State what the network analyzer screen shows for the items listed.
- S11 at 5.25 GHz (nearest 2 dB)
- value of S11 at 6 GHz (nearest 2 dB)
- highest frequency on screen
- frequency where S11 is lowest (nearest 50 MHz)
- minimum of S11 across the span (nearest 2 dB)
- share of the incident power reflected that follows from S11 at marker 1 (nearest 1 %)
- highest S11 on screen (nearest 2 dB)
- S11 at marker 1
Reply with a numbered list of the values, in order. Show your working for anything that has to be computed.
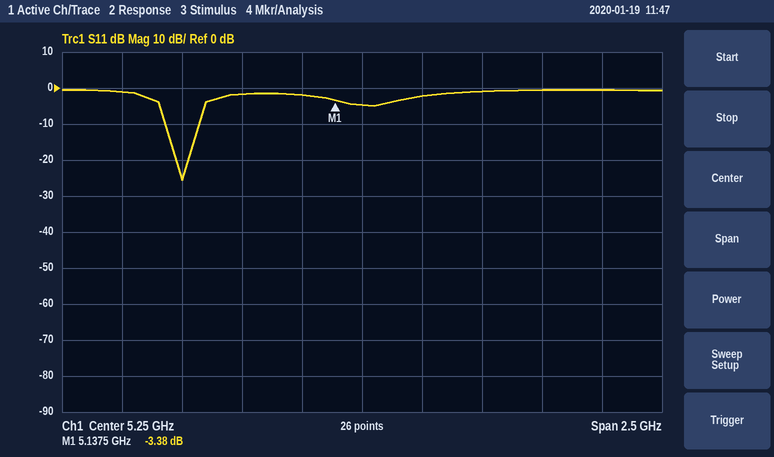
1. -4 dB
2. 0 dB
3. 6.5 GHz
4. 4.50 GHz
5. -26 dB
6. 10^(-3.38/10) ≈ 46 %
7. 0 dB
8. -3.38 dB
